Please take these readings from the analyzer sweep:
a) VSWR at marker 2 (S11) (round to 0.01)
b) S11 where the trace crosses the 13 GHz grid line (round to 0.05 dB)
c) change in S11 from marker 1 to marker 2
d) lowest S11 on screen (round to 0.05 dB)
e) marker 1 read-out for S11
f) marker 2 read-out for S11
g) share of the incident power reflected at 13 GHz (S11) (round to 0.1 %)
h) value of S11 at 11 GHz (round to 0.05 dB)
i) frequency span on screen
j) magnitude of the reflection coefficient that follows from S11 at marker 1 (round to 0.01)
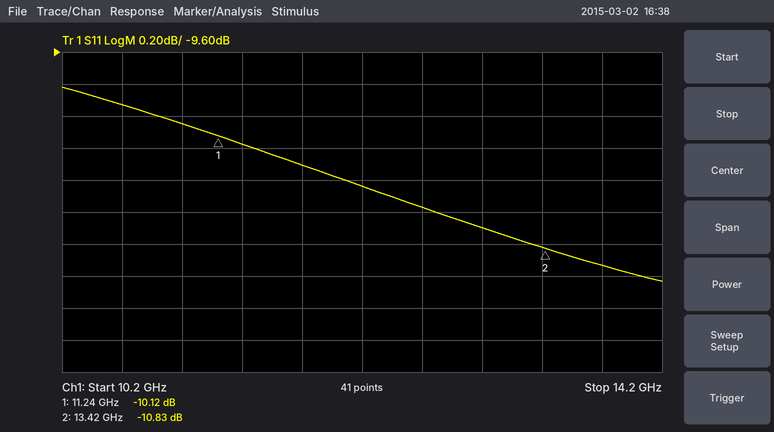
1.81
-10.70 dB
-0.71 dB
-11.05 dB
-10.12 dB
-10.83 dB
8.5 %
-10.05 dB
4 GHz
0.31
